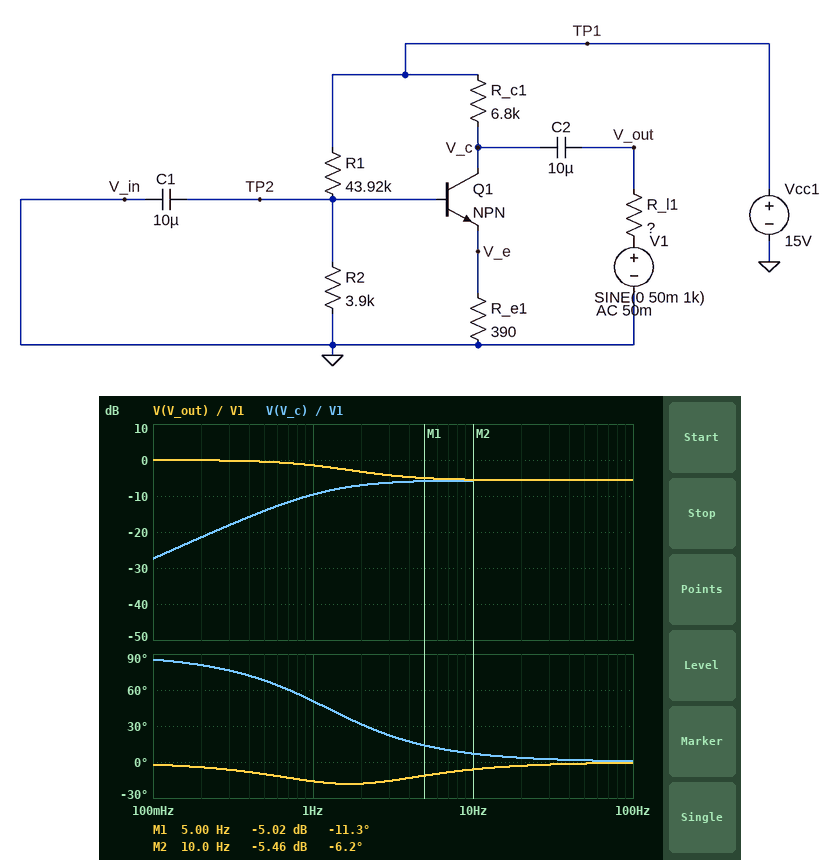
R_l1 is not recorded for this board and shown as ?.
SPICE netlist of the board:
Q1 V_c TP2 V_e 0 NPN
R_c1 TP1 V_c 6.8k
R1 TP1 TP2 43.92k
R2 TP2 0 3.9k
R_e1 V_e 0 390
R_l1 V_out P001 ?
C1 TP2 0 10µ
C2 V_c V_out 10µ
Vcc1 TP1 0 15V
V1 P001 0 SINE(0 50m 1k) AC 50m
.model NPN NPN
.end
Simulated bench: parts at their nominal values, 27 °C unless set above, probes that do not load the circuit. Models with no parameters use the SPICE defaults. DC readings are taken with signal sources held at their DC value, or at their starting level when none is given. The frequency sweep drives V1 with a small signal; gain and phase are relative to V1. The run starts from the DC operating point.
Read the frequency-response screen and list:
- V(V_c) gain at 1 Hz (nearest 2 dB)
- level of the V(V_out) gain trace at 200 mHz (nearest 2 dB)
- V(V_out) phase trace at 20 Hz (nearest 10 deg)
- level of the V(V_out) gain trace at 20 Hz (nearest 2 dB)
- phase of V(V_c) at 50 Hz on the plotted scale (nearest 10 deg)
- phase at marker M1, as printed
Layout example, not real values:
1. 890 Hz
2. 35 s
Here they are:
1. -10 dB
2. 0 dB
3. 0 deg
4. -6 dB
5. 0 deg
6. -11.3 deg
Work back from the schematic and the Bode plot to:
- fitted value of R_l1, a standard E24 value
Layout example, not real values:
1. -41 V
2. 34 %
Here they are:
1. 6.2 kΩ
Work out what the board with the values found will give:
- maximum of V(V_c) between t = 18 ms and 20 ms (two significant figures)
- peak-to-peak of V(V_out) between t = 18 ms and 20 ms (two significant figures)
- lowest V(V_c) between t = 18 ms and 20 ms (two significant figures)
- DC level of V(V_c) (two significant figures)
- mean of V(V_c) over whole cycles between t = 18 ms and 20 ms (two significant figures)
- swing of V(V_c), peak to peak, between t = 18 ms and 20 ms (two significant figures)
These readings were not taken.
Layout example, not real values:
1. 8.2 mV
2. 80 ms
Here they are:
1. 7.9 V
2. 52 mV
3. 7.9 V
4. 7.9 V
5. 7.9 V
6. 52 mV
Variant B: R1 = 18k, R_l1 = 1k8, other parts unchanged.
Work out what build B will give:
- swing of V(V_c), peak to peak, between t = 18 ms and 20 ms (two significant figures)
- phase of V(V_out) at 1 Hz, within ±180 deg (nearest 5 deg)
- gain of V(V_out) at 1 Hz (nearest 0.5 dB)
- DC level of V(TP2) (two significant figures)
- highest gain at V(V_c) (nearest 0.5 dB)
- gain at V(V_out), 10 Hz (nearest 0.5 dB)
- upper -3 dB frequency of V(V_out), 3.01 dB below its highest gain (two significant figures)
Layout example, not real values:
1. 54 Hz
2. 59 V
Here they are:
1. 4.9 mV
2. -5 deg
3. 0 dB
4. 1.7 V
5. -17.0 dB
6. -4.0 dB
7. 7.8 Hz
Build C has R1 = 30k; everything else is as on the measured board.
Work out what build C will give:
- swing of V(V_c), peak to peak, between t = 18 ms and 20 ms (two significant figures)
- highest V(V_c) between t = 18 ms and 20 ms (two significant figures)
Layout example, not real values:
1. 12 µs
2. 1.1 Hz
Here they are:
1. 21 mV
2. 960 mV
